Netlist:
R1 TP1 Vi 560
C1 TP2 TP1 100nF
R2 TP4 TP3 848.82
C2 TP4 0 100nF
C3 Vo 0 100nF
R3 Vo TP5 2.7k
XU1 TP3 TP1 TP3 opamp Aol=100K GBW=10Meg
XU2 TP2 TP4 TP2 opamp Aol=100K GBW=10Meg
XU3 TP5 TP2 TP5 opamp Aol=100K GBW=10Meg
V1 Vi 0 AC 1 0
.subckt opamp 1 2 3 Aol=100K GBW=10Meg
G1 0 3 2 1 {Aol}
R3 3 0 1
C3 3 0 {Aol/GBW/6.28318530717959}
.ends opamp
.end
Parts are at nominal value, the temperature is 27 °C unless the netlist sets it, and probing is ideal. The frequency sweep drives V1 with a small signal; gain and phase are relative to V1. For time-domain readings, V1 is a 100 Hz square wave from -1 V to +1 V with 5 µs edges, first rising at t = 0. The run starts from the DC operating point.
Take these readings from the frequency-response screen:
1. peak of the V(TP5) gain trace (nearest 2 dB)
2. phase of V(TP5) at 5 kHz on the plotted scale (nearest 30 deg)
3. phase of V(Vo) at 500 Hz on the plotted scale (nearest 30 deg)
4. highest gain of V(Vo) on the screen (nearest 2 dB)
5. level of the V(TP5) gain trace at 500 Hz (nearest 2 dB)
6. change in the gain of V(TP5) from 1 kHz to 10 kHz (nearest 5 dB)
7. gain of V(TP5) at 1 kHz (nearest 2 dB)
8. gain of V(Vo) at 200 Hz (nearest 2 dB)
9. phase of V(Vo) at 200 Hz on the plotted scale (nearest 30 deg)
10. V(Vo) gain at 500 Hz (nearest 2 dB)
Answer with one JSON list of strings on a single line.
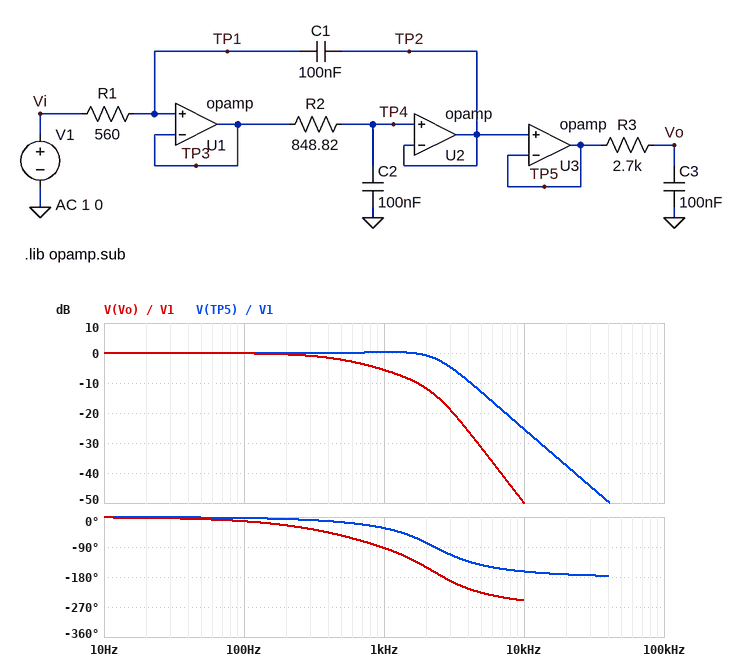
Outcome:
["0 dB", "-150 deg", "-60 deg", "0 dB", "0 dB", "-25 dB", "0 dB", "0 dB", "-30 deg", "-2 dB"]
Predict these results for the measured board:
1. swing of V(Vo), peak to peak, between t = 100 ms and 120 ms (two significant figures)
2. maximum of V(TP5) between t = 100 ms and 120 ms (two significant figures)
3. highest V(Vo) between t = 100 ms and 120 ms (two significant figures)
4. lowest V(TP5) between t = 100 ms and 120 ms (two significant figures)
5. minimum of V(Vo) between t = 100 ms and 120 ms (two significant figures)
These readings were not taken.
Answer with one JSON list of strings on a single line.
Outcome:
["2.0 V", "1.2 V", "1.0 V", "-1.2 V", "-1.0 V"]
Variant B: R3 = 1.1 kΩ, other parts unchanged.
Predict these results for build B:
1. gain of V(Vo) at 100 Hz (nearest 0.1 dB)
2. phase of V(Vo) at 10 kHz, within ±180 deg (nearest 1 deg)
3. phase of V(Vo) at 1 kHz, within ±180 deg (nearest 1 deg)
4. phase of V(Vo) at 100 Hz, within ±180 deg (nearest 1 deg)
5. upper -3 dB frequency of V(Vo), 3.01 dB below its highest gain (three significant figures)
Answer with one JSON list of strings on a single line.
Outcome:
["0 dB", "115 deg", "-68 deg", "-7 deg", "1.49 kHz"]
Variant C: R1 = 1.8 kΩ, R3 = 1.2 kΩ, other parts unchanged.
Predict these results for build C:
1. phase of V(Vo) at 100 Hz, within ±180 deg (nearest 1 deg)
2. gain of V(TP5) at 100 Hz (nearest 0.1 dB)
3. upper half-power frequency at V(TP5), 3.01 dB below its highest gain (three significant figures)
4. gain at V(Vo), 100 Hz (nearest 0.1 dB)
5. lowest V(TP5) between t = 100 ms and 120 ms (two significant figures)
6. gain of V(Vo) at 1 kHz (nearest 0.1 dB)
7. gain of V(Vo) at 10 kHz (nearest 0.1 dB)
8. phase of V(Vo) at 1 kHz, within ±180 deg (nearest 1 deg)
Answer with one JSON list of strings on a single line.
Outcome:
["-7 deg", "0 dB", "1.53 kHz", "0 dB", "-1.6 V", "1.6 dB", "-53.1 dB", "-90 deg"]
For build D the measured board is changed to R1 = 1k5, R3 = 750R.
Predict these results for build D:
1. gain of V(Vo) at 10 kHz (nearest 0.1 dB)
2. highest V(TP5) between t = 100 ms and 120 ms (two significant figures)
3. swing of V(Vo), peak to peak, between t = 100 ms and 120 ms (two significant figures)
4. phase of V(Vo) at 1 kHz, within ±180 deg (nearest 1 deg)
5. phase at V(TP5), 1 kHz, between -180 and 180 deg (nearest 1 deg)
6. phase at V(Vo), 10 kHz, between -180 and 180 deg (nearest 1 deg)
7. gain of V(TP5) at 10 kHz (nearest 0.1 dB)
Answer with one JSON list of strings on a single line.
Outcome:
["-47.6 dB", "1.6 V", "2.9 V", "-72 deg", "-47 deg", "108 deg", "-33.9 dB"]
